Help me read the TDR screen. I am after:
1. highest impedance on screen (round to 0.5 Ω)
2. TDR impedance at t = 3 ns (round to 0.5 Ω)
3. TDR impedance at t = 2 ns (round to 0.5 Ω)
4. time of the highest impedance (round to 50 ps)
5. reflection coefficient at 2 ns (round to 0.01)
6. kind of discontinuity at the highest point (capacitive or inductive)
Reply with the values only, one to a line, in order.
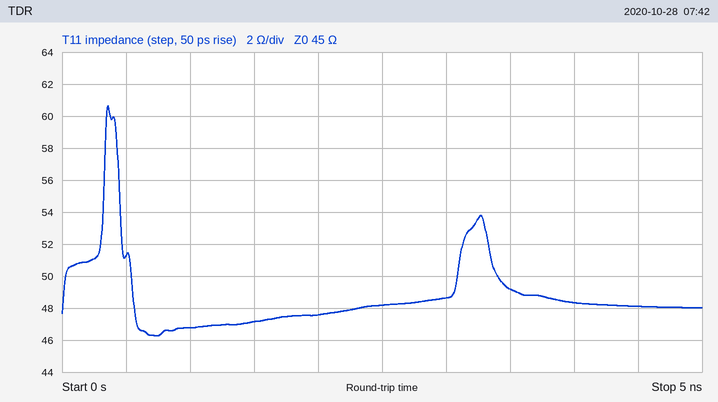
60.5 Ω
48.5 Ω
47.5 Ω
350 ps
+0.03
inductive
